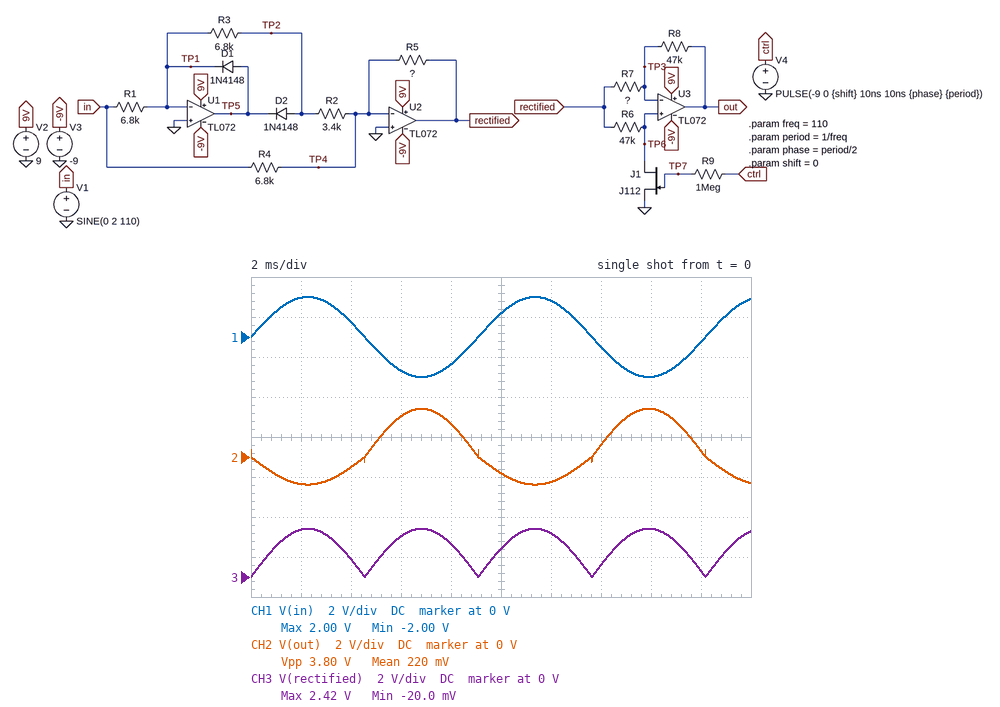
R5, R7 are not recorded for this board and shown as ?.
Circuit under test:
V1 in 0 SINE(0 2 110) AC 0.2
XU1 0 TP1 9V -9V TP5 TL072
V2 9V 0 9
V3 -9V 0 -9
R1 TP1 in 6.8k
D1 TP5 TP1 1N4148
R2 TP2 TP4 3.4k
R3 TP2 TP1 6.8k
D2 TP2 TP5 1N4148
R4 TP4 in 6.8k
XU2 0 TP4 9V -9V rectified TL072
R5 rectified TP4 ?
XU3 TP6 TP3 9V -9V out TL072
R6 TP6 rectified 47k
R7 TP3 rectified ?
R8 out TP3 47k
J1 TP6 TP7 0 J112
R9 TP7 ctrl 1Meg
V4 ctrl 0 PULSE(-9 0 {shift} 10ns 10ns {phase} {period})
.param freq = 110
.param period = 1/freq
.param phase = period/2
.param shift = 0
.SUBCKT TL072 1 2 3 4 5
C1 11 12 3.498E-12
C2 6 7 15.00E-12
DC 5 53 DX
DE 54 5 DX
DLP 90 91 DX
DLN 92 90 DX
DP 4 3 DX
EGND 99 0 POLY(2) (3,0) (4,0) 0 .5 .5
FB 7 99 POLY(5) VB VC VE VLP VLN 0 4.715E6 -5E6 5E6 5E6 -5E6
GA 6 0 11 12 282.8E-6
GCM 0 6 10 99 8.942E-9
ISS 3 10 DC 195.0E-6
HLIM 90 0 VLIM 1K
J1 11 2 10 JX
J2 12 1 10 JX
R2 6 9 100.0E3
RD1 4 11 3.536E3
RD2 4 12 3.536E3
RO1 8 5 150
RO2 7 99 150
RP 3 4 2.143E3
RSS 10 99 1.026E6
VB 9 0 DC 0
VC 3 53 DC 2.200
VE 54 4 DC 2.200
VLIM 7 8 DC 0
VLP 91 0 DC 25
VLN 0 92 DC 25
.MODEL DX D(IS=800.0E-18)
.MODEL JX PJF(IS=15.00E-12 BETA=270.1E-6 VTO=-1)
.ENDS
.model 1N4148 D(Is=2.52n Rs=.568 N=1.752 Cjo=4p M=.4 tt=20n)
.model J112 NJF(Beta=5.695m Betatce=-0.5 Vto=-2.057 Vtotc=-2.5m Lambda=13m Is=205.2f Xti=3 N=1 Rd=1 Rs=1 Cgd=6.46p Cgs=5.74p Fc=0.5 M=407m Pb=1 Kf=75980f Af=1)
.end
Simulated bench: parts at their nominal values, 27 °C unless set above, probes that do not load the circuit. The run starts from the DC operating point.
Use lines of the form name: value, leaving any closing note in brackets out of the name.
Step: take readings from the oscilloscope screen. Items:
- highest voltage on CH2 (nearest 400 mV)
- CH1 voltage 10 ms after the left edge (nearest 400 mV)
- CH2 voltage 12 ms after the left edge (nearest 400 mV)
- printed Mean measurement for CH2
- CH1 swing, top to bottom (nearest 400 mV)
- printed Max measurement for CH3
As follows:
highest voltage on CH2: 2.4 V
CH1 voltage 10 ms after the left edge: 1.2 V
CH2 voltage 12 ms after the left edge: -1.2 V
printed Mean measurement for CH2: 220 mV
CH1 swing, top to bottom: 4.0 V
printed Max measurement for CH3: 2.42 V
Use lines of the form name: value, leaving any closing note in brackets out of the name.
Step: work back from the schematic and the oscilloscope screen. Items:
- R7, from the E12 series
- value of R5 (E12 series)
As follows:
R7, from the E12 series: 82 kΩ
value of R5: 8.2 kΩ
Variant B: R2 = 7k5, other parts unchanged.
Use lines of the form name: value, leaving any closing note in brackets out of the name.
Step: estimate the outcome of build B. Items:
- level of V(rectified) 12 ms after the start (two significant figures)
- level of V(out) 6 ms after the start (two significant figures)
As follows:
level of V(rectified) 12 ms after the start: -200 mV
level of V(out) 6 ms after the start: 2.0 V
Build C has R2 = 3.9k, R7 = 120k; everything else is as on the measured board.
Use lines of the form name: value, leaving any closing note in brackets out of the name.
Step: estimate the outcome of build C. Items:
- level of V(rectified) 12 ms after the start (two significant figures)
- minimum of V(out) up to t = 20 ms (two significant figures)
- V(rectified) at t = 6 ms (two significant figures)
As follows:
level of V(rectified) 12 ms after the start: 1.6 V
minimum of V(out) up to t = 20 ms: -700 mV
V(rectified) at t = 6 ms: 2.0 V
